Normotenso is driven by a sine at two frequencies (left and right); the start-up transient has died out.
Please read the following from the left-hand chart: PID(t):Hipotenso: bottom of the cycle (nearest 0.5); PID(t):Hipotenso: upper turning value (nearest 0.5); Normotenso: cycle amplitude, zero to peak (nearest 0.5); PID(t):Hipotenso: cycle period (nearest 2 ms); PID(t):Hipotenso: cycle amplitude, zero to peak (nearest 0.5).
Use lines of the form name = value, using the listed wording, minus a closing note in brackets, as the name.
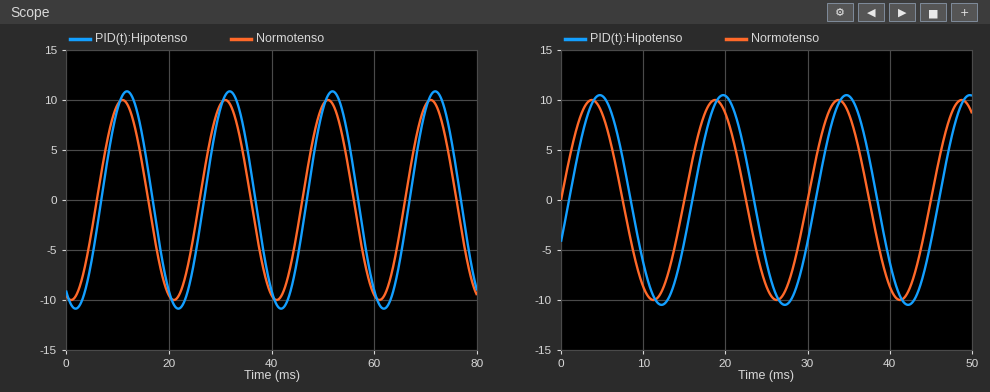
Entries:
PID(t):Hipotenso: bottom of the cycle = -11.0
PID(t):Hipotenso: upper turning value = 11.0
Normotenso: cycle amplitude, zero to peak = 10.0
PID(t):Hipotenso: cycle period = 20 ms
PID(t):Hipotenso: cycle amplitude, zero to peak = 11.0
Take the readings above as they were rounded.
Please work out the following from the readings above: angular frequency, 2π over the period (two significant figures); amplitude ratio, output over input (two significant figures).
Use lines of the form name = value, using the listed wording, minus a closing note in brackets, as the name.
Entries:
angular frequency, 2π over the period = 0.31 rad/ms
amplitude ratio, output over input = 1.1
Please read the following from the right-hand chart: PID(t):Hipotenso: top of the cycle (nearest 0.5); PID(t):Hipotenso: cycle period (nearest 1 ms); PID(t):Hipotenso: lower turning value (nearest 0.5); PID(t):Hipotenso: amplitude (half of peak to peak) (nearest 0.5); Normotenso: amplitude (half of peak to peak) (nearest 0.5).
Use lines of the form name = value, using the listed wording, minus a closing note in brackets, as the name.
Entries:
PID(t):Hipotenso: top of the cycle = 10.5
PID(t):Hipotenso: cycle period = 15 ms
PID(t):Hipotenso: lower turning value = -10.5
PID(t):Hipotenso: amplitude (half of peak to peak) = 10.5
Normotenso: amplitude (half of peak to peak) = 10.0
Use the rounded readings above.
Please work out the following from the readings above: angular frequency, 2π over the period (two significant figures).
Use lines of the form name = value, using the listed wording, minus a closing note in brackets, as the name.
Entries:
angular frequency, 2π over the period = 0.42 rad/ms
